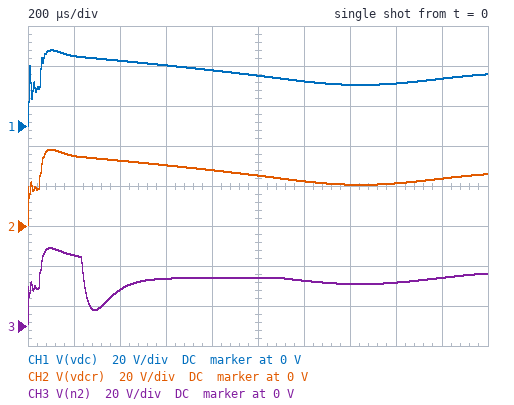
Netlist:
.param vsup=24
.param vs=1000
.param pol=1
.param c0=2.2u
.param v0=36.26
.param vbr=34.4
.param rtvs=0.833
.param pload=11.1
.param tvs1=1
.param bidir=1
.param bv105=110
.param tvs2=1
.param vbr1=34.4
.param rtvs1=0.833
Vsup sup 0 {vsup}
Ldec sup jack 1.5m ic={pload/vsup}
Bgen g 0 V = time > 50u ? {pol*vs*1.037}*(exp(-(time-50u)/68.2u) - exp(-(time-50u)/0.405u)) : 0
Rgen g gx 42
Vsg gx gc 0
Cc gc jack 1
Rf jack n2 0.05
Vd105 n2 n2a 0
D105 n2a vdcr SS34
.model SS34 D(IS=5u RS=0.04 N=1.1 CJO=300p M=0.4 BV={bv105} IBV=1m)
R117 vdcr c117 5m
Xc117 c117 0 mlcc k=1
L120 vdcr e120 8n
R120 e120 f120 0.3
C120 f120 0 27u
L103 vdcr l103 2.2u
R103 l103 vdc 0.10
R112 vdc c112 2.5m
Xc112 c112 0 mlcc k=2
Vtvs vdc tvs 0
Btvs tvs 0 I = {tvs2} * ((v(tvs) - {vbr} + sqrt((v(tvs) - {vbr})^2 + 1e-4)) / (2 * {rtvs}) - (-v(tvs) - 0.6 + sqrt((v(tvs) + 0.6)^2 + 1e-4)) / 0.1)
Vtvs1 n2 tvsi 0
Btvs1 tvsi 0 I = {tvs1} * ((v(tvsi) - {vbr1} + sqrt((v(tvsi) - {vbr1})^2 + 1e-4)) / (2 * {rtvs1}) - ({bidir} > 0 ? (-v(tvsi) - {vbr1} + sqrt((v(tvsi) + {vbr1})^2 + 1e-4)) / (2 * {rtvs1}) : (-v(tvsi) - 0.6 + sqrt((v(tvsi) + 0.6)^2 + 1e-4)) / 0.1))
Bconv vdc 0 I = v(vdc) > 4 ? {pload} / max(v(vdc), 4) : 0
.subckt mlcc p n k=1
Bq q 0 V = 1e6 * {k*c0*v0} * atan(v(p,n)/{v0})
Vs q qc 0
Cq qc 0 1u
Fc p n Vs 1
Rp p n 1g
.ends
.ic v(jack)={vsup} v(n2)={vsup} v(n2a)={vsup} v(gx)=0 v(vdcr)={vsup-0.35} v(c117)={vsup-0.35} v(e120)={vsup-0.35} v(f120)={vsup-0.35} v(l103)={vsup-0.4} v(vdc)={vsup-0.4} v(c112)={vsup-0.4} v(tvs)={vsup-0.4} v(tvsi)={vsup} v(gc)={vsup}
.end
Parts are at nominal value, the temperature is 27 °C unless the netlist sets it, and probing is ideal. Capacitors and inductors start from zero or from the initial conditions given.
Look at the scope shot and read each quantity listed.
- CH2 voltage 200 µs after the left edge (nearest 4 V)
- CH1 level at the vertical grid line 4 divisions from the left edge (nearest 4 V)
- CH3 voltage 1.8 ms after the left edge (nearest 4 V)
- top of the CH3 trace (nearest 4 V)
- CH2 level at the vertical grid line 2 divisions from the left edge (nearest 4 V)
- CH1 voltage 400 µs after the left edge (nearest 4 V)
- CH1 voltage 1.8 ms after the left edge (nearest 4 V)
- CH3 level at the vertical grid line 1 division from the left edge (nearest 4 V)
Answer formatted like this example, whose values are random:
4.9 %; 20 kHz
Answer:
36 V; 28 V; 24 V; 40 V; 32 V; 32 V; 24 V; 36 V
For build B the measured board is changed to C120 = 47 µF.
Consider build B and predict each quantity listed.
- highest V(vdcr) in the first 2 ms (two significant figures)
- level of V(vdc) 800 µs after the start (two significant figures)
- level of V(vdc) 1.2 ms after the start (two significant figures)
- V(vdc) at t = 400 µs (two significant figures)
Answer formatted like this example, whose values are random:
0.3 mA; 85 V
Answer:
37 V; 31 V; 28 V; 34 V
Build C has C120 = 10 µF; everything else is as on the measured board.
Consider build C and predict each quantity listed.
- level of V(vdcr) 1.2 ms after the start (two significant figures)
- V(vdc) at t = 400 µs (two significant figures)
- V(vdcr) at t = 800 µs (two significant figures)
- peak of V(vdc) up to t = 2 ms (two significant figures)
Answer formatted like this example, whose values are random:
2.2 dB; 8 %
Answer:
27 V; 30 V; 19 V; 40 V
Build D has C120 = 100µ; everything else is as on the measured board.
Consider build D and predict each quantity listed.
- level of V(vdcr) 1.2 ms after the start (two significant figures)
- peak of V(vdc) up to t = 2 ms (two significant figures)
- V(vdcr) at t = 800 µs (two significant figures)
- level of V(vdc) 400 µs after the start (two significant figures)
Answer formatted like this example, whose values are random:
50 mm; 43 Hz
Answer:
31 V; 35 V; 32 V; 34 V
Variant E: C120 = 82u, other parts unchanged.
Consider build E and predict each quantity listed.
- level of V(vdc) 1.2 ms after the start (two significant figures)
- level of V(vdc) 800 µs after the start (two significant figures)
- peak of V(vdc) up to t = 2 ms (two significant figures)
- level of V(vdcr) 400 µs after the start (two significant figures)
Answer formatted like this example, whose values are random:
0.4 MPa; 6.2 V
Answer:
31 V; 32 V; 35 V; 34 V
